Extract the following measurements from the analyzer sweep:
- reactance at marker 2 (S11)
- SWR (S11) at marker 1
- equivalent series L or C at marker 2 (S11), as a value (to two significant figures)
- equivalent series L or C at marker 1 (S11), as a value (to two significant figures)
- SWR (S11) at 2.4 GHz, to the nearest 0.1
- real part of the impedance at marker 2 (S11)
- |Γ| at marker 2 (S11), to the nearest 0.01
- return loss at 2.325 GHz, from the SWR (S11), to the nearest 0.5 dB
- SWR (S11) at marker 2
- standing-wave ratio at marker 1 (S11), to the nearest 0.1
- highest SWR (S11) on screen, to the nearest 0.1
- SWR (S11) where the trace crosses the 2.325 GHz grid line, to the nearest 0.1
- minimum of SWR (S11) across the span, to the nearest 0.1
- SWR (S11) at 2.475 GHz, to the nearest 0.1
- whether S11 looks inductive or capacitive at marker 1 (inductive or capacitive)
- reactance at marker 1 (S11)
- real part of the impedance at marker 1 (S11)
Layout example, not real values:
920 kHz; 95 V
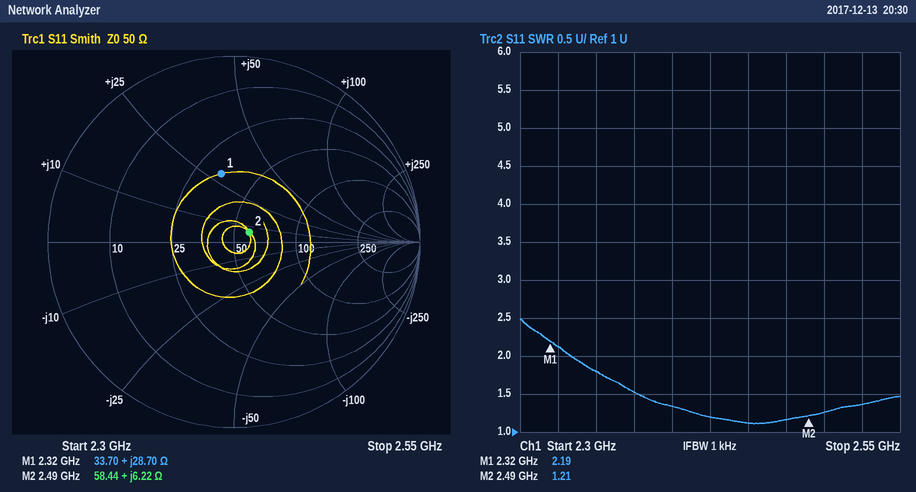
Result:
+6.22 Ω; 2.19; 400 pH; 2.0 nH; 1.3; 58.44 Ω; 0.10; 9.0 dB; 1.21; 2.2; 2.5; 2.1; 1.1; 1.2; inductive; +28.70 Ω; 33.70 Ω
